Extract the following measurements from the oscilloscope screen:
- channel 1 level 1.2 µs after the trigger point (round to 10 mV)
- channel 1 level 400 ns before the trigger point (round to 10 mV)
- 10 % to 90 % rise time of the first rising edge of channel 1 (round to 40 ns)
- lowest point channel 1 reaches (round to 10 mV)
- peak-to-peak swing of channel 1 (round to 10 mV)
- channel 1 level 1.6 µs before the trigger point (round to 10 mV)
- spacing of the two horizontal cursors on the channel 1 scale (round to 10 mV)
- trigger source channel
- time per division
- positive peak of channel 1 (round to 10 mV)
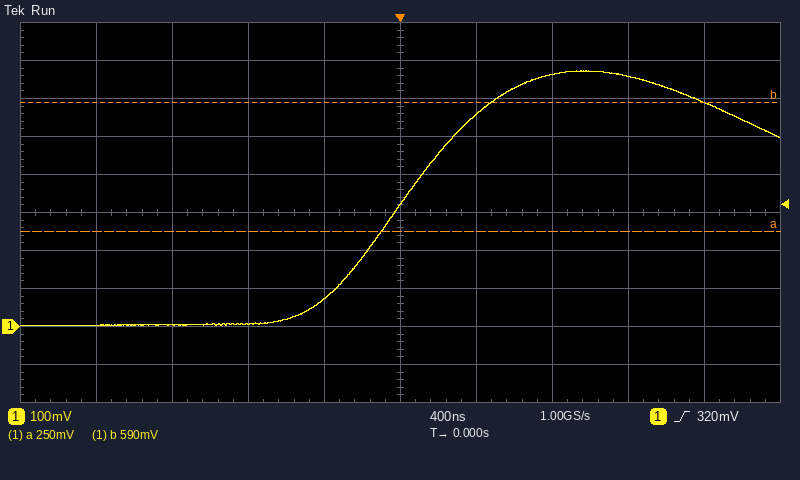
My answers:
660 mV
70 mV
920 ns
0 mV
670 mV
0 mV
340 mV
channel 1
400 ns
670 mV
